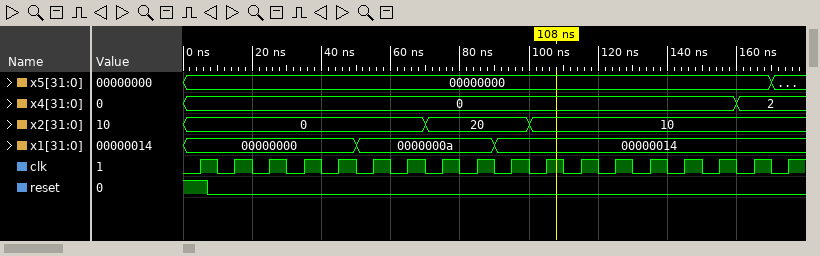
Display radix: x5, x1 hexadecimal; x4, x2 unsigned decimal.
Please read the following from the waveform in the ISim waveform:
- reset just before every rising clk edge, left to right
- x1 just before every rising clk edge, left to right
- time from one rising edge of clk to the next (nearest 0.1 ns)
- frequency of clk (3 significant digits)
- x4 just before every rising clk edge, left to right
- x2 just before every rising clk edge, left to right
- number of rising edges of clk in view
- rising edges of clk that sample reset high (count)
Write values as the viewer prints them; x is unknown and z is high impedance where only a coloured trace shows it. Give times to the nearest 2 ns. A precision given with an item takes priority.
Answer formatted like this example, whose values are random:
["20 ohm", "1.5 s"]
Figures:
["1 0 0 0 0 0 0 0 0 0 0 0 0 0 0 0 0 0", "00000000, 00000000, 00000000, 00000000, 00000000, 0000000a, 0000000a, 0000000a, 0000000a, 00000014, 00000014, 00000014, 00000014, 00000014, 00000014, 00000014, 00000014, 00000014", "10 ns", "100 MHz", "0, 0, 0, 0, 0, 0, 0, 0, 0, 0, 0, 0, 0, 0, 0, 0, 2, 2", "0, 0, 0, 0, 0, 0, 0, 20, 20, 20, 10, 10, 10, 10, 10, 10, 10, 10", "18", "1"]
